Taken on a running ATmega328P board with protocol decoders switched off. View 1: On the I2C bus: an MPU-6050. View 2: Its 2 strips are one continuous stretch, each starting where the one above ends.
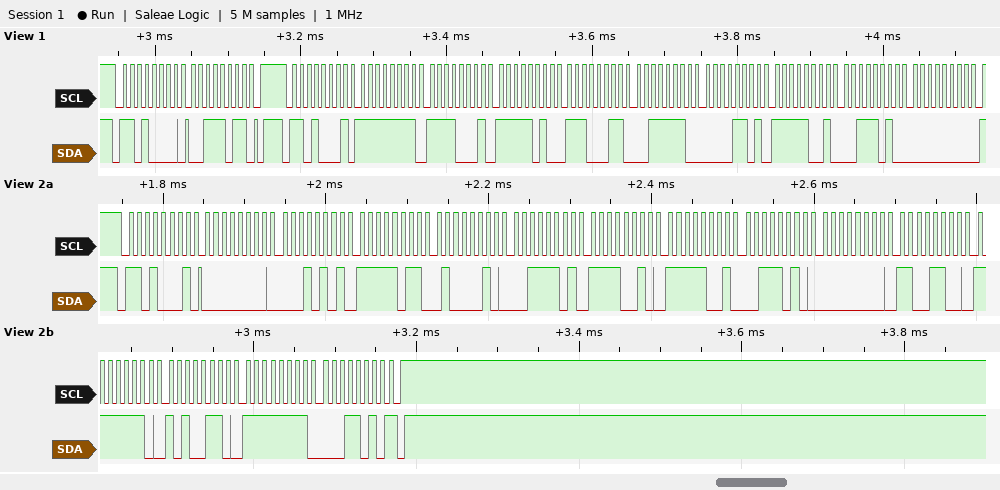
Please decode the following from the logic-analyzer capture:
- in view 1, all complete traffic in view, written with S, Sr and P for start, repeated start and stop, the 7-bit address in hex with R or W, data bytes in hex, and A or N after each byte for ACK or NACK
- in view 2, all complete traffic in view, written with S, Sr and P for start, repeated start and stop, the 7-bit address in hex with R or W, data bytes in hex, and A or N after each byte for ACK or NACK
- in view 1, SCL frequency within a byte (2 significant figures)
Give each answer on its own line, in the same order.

S 68W A 3B A P S 68R A FF A F1 A FA A E3 A 3E A 0D A F9 A 3A A 00 A
S 68R A 00 A 15 A FB A 42 A 3D A F2 A F9 A 3A A 00 A CC A FE A A6 A FF A 1A N P
100 kHz
